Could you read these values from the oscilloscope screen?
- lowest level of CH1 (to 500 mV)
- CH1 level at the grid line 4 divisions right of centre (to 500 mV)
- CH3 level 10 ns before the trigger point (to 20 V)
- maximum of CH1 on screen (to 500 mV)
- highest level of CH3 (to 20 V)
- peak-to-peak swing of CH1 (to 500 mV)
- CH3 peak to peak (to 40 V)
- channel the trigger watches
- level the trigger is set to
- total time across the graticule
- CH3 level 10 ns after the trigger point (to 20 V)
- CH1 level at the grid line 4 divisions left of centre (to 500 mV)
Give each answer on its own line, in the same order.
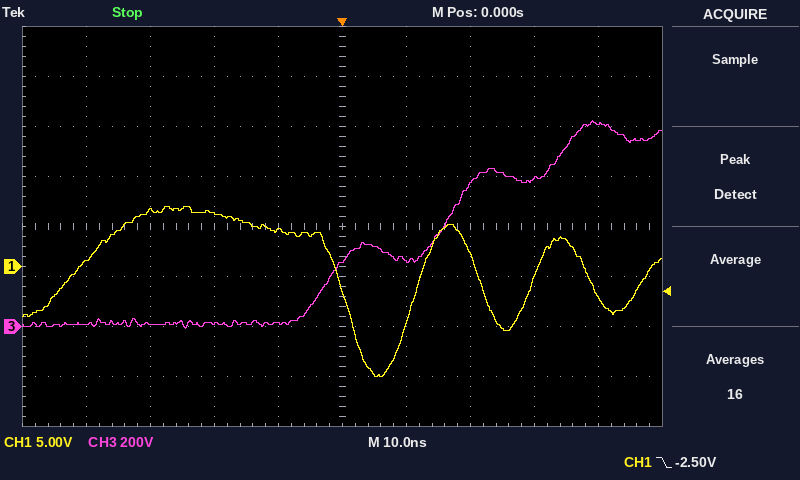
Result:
-11.0 V
-3.0 V
20 V
6.0 V
820 V
17.0 V
840 V
CH1
-2.50 V
100 ns
260 V
500 mV
